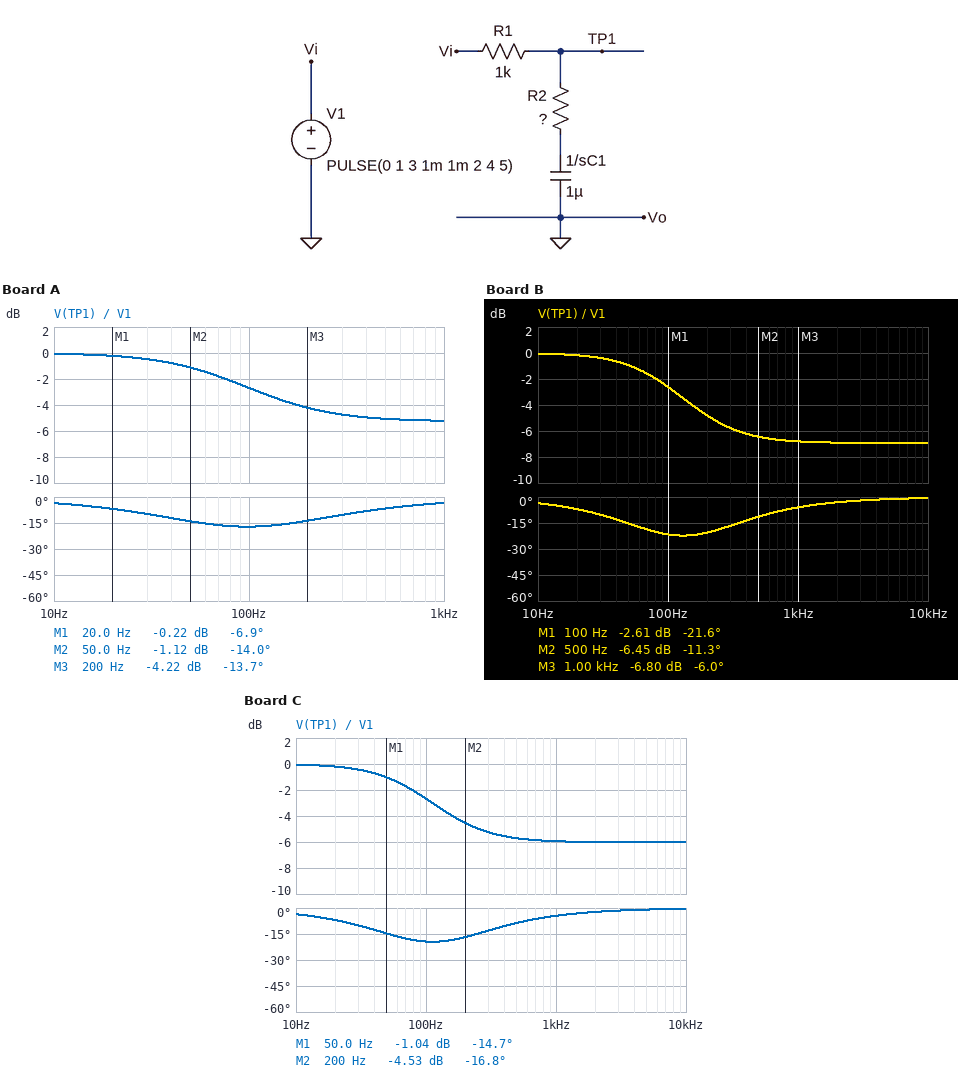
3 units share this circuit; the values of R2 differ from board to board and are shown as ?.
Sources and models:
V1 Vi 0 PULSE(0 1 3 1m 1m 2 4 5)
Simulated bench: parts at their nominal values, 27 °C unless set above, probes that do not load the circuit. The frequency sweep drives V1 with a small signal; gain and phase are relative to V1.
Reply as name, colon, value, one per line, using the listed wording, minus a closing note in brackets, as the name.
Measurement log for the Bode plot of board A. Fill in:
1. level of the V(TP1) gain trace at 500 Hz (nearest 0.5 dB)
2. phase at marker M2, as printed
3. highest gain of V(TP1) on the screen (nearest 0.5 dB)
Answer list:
level of the V(TP1) gain trace at 500 Hz: -5.0 dB
phase at marker M2, as printed: -14.0 deg
highest gain of V(TP1) on the screen: 0 dB
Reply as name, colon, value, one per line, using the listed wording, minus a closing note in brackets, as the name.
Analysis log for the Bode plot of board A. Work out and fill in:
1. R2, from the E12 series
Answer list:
R2, from the E12 series: 1.2 kΩ
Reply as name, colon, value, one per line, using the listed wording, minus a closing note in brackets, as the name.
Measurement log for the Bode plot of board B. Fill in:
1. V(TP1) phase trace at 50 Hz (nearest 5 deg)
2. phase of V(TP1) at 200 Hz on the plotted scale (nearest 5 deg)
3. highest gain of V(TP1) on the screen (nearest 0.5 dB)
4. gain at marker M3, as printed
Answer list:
V(TP1) phase trace at 50 Hz: -15 deg
phase of V(TP1) at 200 Hz on the plotted scale: -20 deg
highest gain of V(TP1) on the screen: 0 dB
gain at marker M3, as printed: -6.80 dB
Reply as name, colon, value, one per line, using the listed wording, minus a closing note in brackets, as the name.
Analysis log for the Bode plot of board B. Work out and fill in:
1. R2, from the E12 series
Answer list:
R2, from the E12 series: 820 Ω
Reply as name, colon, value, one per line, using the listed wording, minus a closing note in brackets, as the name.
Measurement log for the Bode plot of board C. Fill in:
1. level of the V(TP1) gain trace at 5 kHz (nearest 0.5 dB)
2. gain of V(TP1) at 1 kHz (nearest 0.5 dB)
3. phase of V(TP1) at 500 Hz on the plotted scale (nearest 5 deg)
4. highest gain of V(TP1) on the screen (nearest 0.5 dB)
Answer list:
level of the V(TP1) gain trace at 5 kHz: -6.0 dB
gain of V(TP1) at 1 kHz: -6.0 dB
phase of V(TP1) at 500 Hz on the plotted scale: -10 deg
highest gain of V(TP1) on the screen: 0 dB
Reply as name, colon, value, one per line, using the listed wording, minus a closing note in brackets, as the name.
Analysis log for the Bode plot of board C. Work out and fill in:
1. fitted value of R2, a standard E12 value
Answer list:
fitted value of R2, a standard E12 value: 1 kΩ
